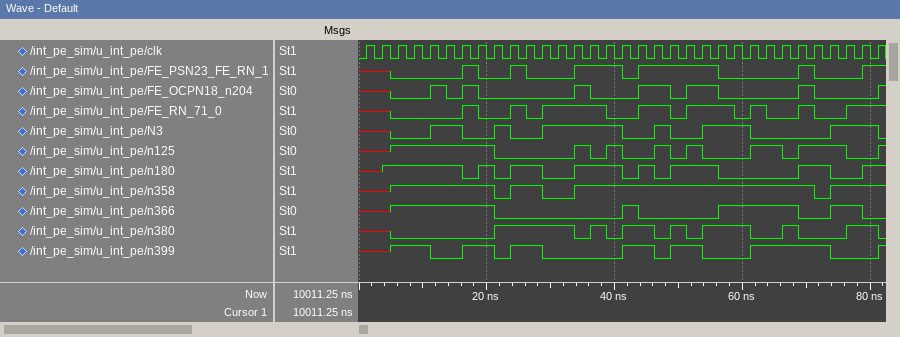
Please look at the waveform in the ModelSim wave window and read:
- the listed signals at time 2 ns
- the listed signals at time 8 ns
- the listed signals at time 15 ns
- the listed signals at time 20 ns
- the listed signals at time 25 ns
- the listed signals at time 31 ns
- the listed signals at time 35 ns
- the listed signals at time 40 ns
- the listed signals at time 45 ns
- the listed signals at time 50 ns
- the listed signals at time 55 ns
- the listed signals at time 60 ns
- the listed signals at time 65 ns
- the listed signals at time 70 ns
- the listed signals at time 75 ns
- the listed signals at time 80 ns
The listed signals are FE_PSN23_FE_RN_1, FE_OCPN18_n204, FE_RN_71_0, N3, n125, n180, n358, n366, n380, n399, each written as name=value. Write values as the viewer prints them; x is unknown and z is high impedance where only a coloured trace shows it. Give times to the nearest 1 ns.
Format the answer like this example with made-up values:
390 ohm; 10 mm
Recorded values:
FE_PSN23_FE_RN_1=x, FE_OCPN18_n204=x, FE_RN_71_0=x, N3=x, n125=x, n180=x, n358=x, n366=x, n380=x, n399=x; FE_PSN23_FE_RN_1=0, FE_OCPN18_n204=0, FE_RN_71_0=0, N3=0, n125=1, n180=1, n358=1, n366=1, n380=0, n399=1; FE_PSN23_FE_RN_1=0, FE_OCPN18_n204=0, FE_RN_71_0=0, N3=1, n125=1, n180=1, n358=1, n366=1, n380=0, n399=0; FE_PSN23_FE_RN_1=0, FE_OCPN18_n204=0, FE_RN_71_0=0, N3=0, n125=1, n180=1, n358=1, n366=1, n380=0, n399=1; FE_PSN23_FE_RN_1=1, FE_OCPN18_n204=0, FE_RN_71_0=1, N3=0, n125=0, n180=1, n358=1, n366=0, n380=1, n399=1; FE_PSN23_FE_RN_1=0, FE_OCPN18_n204=0, FE_RN_71_0=1, N3=1, n125=0, n180=0, n358=0, n366=0, n380=1, n399=0; FE_PSN23_FE_RN_1=1, FE_OCPN18_n204=1, FE_RN_71_0=1, N3=1, n125=1, n180=1, n358=1, n366=0, n380=0, n399=0; FE_PSN23_FE_RN_1=1, FE_OCPN18_n204=0, FE_RN_71_0=0, N3=1, n125=1, n180=1, n358=1, n366=0, n380=0, n399=0; FE_PSN23_FE_RN_1=1, FE_OCPN18_n204=1, FE_RN_71_0=1, N3=0, n125=0, n180=1, n358=1, n366=0, n380=1, n399=1; FE_PSN23_FE_RN_1=1, FE_OCPN18_n204=0, FE_RN_71_0=0, N3=0, n125=0, n180=1, n358=1, n366=0, n380=1, n399=1; FE_PSN23_FE_RN_1=1, FE_OCPN18_n204=1, FE_RN_71_0=1, N3=1, n125=0, n180=1, n358=1, n366=0, n380=1, n399=0; FE_PSN23_FE_RN_1=0, FE_OCPN18_n204=0, FE_RN_71_0=0, N3=1, n125=0, n180=0, n358=1, n366=1, n380=1, n399=0; FE_PSN23_FE_RN_1=0, FE_OCPN18_n204=0, FE_RN_71_0=0, N3=0, n125=1, n180=0, n358=1, n366=1, n380=0, n399=1; FE_PSN23_FE_RN_1=1, FE_OCPN18_n204=1, FE_RN_71_0=1, N3=0, n125=1, n180=1, n358=1, n366=0, n380=0, n399=1; FE_PSN23_FE_RN_1=0, FE_OCPN18_n204=0, FE_RN_71_0=0, N3=1, n125=1, n180=0, n358=1, n366=1, n380=0, n399=0; FE_PSN23_FE_RN_1=1, FE_OCPN18_n204=0, FE_RN_71_0=1, N3=1, n125=0, n180=1, n358=1, n366=0, n380=1, n399=0
